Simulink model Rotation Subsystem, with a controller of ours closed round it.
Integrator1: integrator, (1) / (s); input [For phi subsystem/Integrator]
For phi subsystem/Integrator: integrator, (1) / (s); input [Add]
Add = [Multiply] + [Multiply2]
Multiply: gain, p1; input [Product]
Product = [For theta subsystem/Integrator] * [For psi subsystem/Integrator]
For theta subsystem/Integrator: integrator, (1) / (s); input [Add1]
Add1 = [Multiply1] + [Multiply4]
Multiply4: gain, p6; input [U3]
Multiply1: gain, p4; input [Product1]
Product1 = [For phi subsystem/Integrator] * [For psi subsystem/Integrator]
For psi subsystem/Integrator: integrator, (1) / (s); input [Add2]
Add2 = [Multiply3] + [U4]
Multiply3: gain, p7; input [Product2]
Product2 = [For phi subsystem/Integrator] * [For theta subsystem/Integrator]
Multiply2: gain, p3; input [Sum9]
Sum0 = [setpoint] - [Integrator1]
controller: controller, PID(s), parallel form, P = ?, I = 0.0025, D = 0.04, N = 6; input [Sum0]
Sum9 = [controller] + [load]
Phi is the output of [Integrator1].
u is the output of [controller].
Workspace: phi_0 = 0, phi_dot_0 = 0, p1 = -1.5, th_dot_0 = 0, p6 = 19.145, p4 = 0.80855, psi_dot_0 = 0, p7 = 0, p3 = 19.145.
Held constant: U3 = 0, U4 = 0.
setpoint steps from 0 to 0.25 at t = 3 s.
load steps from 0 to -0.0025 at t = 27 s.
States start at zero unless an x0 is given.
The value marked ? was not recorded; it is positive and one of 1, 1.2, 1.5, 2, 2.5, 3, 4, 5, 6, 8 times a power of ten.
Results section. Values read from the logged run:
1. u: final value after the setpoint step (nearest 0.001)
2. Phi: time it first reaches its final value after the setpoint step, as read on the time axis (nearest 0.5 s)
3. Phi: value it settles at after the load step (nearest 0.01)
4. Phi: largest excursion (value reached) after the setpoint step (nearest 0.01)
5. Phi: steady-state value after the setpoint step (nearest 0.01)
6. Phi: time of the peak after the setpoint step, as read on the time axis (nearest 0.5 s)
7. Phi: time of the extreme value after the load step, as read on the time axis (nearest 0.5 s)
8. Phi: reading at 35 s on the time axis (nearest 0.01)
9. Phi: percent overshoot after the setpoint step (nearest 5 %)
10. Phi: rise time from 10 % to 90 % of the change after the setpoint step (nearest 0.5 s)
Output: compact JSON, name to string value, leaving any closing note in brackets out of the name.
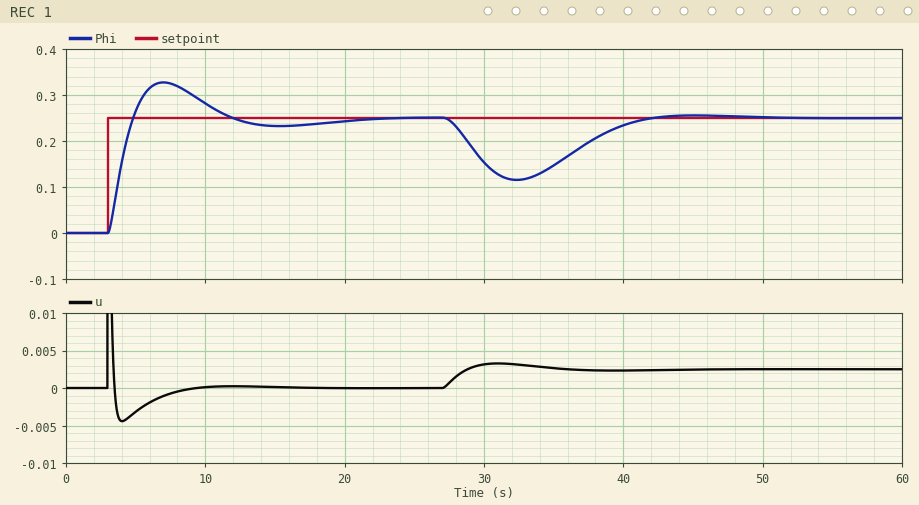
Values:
{"u: final value after the setpoint step": "0.000", "Phi: time it first reaches its final value after the setpoint step, as read on the time axis": "5.0 s", "Phi: value it settles at after the load step": "0.25", "Phi: largest excursion (value reached) after the setpoint step": "0.33", "Phi: steady-state value after the setpoint step": "0.25", "Phi: time of the peak after the setpoint step, as read on the time axis": "7.0 s", "Phi: time of the extreme value after the load step, as read on the time axis": "32.5 s", "Phi: reading at 35 s on the time axis": "0.15", "Phi: percent overshoot after the setpoint step": "30 %", "Phi: rise time from 10 % to 90 % of the change after the setpoint step": "1.5 s"}
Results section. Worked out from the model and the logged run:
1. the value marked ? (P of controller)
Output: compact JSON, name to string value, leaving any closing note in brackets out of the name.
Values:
{"the value marked ?": "0.015"}
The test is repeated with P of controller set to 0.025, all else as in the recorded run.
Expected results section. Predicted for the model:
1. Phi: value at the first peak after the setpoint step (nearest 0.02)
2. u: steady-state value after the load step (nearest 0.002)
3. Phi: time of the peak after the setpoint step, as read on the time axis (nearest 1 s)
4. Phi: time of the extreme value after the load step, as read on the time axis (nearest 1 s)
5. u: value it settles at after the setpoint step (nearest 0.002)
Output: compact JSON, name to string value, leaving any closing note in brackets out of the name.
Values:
{"Phi: value at the first peak after the setpoint step": "0.34", "u: steady-state value after the load step": "0.002", "Phi: time of the peak after the setpoint step, as read on the time axis": "6 s", "Phi: time of the extreme value after the load step, as read on the time axis": "31 s", "u: value it settles at after the setpoint step": "0.000"}
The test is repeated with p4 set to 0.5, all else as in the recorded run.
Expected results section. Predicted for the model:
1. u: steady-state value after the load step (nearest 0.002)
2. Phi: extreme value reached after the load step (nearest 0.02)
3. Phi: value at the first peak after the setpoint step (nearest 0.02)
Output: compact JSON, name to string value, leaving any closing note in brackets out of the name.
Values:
{"u: steady-state value after the load step": "0.002", "Phi: extreme value reached after the load step": "0.12", "Phi: value at the first peak after the setpoint step": "0.32"}
